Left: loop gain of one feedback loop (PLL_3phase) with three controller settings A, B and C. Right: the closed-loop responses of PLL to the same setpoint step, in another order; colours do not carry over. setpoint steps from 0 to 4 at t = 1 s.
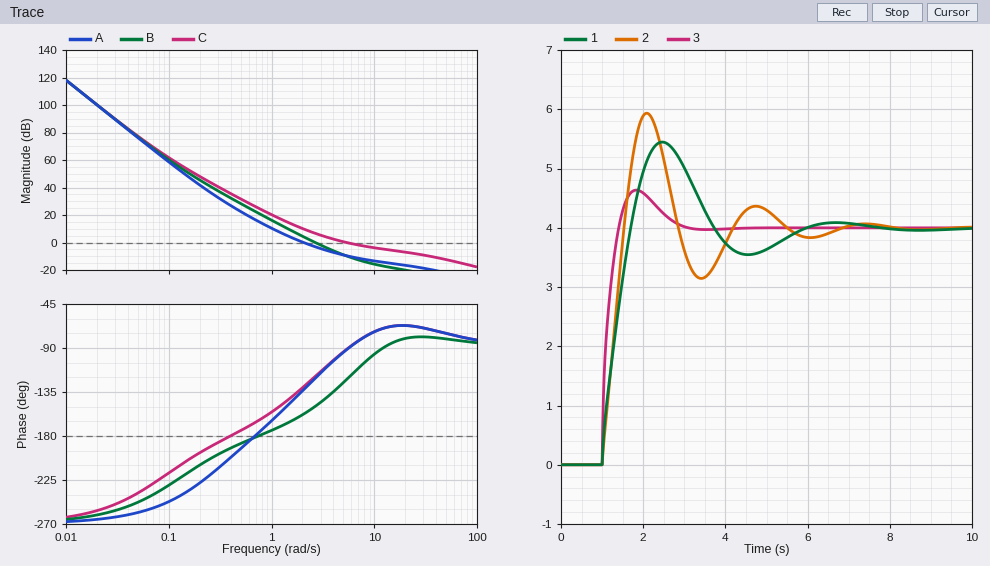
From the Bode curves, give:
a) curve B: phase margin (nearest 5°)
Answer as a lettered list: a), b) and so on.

a) 30°
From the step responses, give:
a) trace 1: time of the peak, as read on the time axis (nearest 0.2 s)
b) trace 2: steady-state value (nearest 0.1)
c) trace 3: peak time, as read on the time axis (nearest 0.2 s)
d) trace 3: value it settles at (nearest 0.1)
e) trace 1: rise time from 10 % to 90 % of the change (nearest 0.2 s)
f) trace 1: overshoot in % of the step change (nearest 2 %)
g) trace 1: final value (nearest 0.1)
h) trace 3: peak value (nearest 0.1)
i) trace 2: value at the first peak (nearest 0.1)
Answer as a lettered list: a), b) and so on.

a) 2.4 s
b) 4.0
c) 1.8 s
d) 4.0
e) 0.6 s
f) 36 %
g) 4.0
h) 4.6
i) 5.9
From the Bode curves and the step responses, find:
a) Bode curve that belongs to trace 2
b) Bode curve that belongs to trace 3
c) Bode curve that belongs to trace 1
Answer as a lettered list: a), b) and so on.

a) B
b) C
c) A
